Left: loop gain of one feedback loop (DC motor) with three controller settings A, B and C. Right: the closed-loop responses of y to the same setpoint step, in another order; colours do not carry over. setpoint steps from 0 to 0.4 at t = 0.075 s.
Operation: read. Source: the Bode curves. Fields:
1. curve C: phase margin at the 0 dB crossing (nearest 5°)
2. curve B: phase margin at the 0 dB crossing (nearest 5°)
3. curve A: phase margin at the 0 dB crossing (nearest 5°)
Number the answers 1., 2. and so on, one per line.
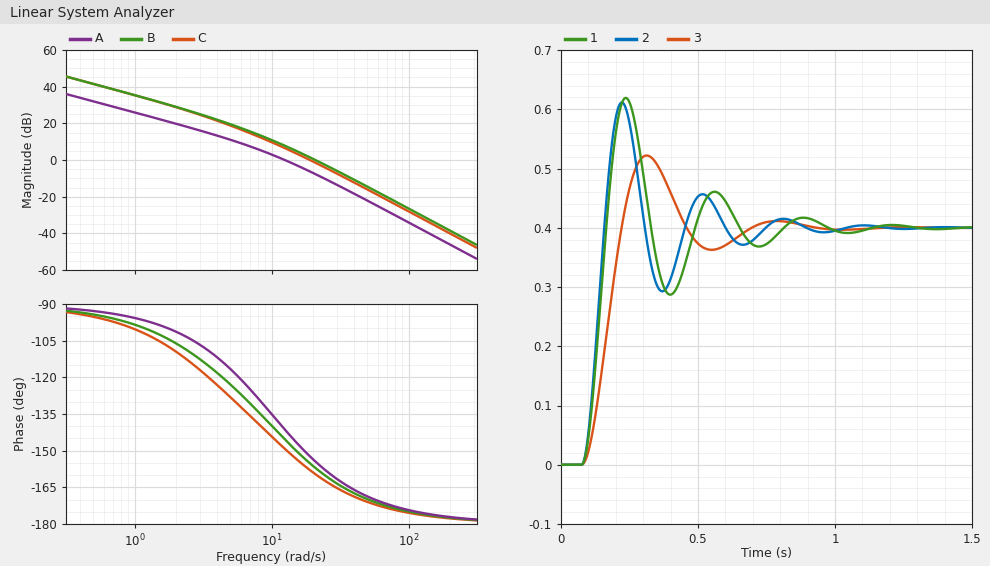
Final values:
1. 20°
2. 25°
3. 40°
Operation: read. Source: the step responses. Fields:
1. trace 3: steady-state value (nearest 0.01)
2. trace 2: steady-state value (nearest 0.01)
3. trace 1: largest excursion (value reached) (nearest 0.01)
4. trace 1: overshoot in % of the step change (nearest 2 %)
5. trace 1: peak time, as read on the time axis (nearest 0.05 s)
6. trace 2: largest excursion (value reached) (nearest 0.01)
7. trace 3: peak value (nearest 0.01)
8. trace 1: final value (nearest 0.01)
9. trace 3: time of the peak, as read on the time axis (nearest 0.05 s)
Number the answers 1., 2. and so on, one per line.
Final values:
1. 0.40
2. 0.40
3. 0.62
4. 54 %
5. 0.25 s
6. 0.61
7. 0.52
8. 0.40
9. 0.30 s
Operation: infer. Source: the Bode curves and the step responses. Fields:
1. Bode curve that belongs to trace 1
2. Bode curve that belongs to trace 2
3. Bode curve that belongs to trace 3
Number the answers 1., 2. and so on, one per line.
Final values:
1. C
2. B
3. A
